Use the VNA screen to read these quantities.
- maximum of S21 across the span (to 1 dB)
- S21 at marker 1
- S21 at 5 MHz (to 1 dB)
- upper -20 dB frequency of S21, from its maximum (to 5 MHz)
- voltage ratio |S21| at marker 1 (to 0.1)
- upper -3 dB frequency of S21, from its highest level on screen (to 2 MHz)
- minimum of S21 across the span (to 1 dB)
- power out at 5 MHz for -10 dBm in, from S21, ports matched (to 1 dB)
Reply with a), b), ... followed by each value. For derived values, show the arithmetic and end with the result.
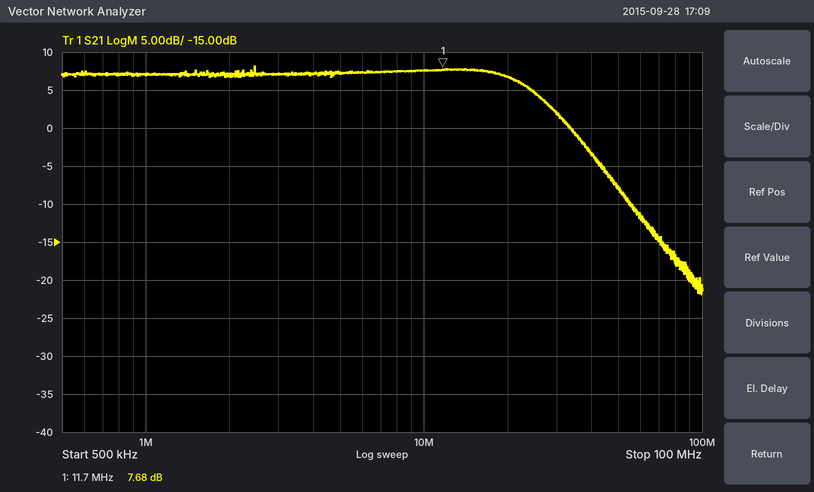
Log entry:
a) 8 dB
b) 7.68 dB
c) 7 dB
d) 60 MHz
e) 10^(7.68/20) ≈ 2.4
f) 24 MHz
g) -22 dB
h) -10 dBm + (7 dB) = -3 dBm
